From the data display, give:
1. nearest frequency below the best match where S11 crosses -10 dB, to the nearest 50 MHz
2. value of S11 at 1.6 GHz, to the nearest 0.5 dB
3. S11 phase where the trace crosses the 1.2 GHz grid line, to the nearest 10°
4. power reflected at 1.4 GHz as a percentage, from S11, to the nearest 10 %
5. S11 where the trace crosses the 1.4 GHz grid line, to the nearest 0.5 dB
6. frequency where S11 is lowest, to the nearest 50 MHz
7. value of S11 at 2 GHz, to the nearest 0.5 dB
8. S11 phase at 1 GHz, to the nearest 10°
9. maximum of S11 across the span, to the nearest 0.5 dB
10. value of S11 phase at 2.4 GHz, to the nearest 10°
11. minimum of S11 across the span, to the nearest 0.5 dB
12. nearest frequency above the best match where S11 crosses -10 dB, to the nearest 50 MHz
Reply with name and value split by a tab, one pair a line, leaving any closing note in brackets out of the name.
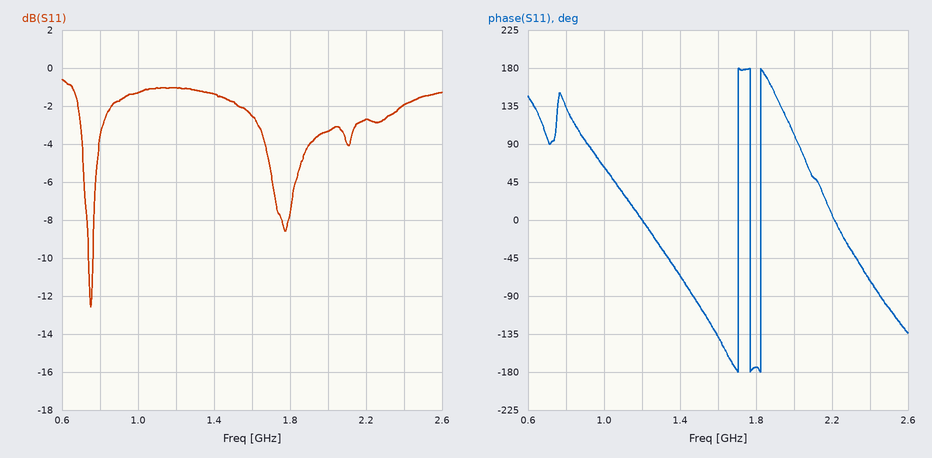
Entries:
nearest frequency below the best match where S11 crosses -10 dB, to the nearest 50 MHz	750 MHz
value of S11 at 1.6 GHz, to the nearest 0.5 dB	-2.5 dB
S11 phase where the trace crosses the 1.2 GHz grid line, to the nearest 10°	0°
power reflected at 1.4 GHz as a percentage, from S11, to the nearest 10 %	70 %
S11 where the trace crosses the 1.4 GHz grid line, to the nearest 0.5 dB	-1.5 dB
frequency where S11 is lowest, to the nearest 50 MHz	750 MHz
value of S11 at 2 GHz, to the nearest 0.5 dB	-3.5 dB
S11 phase at 1 GHz, to the nearest 10°	60°
maximum of S11 across the span, to the nearest 0.5 dB	-0.5 dB
value of S11 phase at 2.4 GHz, to the nearest 10°	-70°
minimum of S11 across the span, to the nearest 0.5 dB	-12.5 dB
nearest frequency above the best match where S11 crosses -10 dB, to the nearest 50 MHz	750 MHz
